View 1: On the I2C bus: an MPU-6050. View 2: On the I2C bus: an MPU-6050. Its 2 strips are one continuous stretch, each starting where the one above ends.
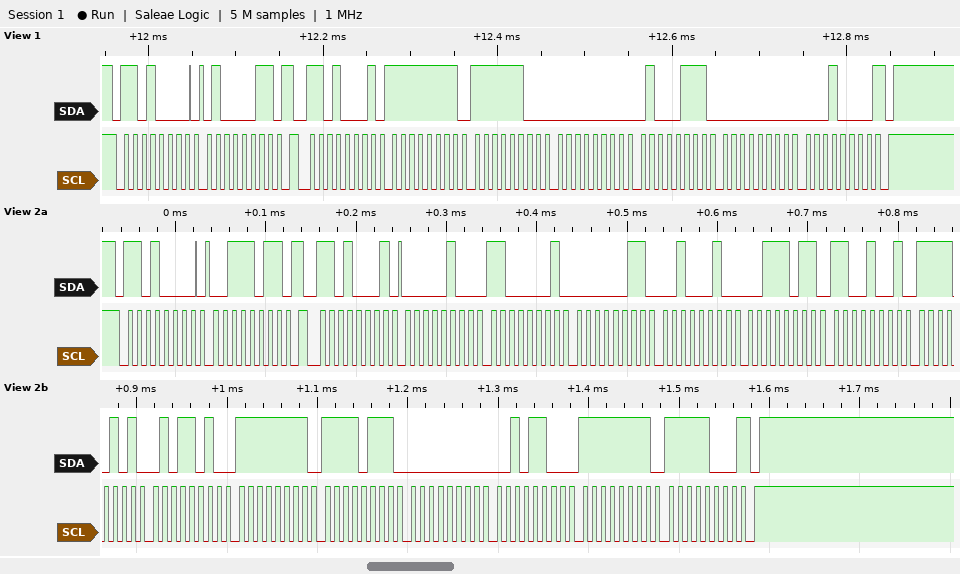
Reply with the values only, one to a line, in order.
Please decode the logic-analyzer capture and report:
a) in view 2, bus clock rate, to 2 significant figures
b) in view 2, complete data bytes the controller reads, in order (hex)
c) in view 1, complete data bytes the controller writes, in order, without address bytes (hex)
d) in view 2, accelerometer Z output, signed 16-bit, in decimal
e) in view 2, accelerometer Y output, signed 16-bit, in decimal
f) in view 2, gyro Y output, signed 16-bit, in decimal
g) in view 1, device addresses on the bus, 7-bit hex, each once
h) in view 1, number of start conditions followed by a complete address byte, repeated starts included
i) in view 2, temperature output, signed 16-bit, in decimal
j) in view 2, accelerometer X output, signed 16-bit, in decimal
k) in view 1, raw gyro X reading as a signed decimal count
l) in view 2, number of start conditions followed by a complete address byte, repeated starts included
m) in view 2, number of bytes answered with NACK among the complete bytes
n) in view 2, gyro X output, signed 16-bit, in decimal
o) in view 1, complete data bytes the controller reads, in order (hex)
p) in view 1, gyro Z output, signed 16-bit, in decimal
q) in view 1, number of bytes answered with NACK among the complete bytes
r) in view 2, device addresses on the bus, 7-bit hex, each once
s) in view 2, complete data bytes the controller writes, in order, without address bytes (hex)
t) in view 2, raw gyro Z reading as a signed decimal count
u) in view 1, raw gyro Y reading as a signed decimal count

100 kHz
04 C1 03 22 3B C9 F5 5A FF F7 00 2C FF F8
43
15305
802
44
0x68
2
-2726
1217
-4
2
1
-9
FF FC 00 47 00 10
16
1
0x68
3B
-8
71
